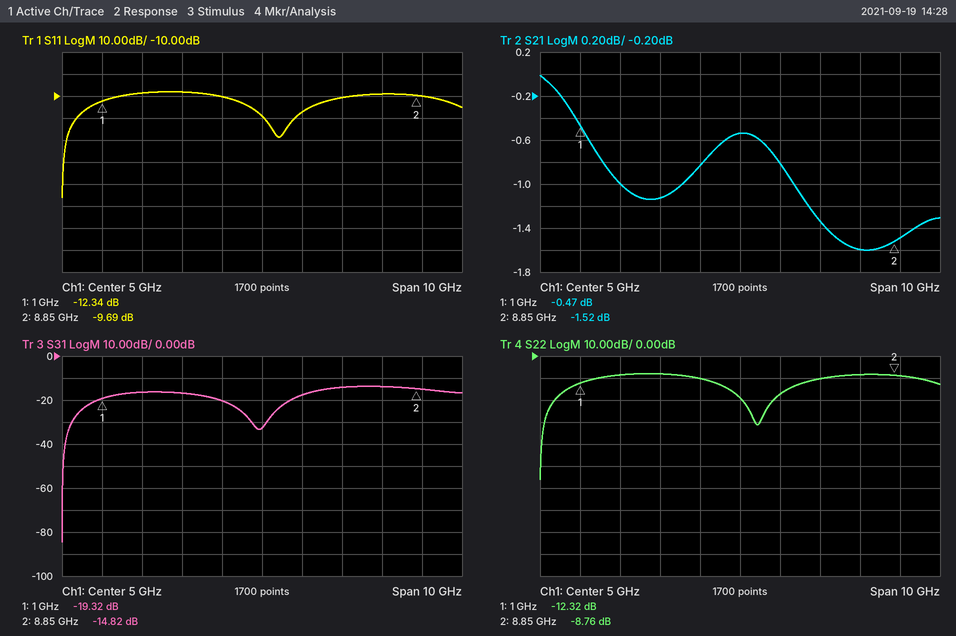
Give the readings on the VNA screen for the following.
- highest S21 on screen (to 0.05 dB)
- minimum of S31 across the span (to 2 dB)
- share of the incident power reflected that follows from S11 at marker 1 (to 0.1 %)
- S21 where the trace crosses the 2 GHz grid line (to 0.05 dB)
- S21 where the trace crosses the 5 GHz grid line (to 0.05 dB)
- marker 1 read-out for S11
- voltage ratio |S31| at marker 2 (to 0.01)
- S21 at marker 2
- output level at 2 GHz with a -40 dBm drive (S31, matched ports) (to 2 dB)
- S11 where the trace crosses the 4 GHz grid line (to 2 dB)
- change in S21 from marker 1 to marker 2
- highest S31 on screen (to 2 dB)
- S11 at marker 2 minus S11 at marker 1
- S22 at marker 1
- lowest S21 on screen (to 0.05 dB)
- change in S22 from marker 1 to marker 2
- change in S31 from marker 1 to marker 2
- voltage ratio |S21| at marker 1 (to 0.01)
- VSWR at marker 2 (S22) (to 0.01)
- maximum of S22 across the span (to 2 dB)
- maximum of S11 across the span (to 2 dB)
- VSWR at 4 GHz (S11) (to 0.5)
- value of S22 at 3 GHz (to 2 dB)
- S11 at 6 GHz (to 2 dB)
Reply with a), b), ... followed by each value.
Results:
a) 0.00 dB
b) -84 dB
c) 5.8 %
d) -1.00 dB
e) -0.55 dB
f) -12.34 dB
g) 0.18
h) -1.52 dB
i) -56 dBm
j) -10 dB
k) -1.05 dB
l) -14 dB
m) 2.65 dB
n) -12.32 dB
o) -1.60 dB
p) 3.56 dB
q) 4.50 dB
r) 0.95
s) 2.15
t) -8 dB
u) -8 dB
v) 2.0
w) -8 dB
x) -18 dB
